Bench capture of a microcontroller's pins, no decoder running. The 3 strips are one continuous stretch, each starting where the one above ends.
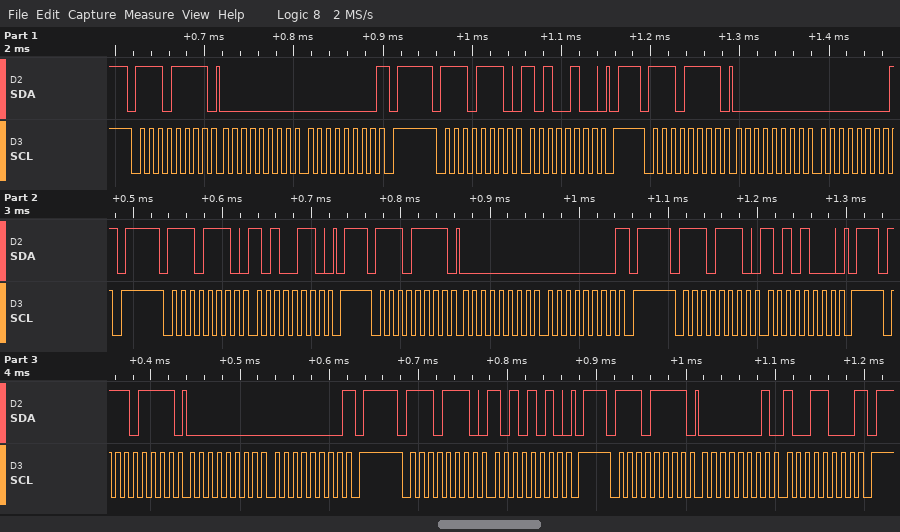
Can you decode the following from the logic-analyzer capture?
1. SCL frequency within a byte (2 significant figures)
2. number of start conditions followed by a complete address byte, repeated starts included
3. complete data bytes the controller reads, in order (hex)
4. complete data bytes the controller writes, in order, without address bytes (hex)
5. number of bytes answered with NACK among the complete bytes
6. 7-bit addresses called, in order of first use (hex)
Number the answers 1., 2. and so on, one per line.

1. 100 kHz
2. 9
3. 00 00 00 00 00 00 00 00 01 98
4. A4 A6 A8 AA
5. 5
6. 0x77
